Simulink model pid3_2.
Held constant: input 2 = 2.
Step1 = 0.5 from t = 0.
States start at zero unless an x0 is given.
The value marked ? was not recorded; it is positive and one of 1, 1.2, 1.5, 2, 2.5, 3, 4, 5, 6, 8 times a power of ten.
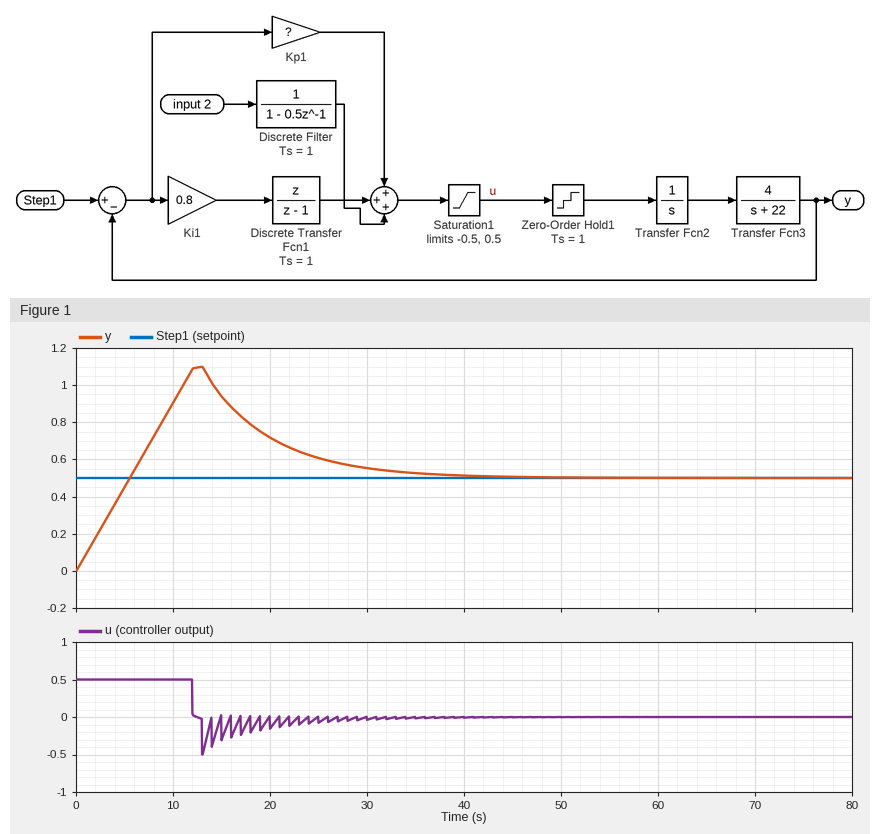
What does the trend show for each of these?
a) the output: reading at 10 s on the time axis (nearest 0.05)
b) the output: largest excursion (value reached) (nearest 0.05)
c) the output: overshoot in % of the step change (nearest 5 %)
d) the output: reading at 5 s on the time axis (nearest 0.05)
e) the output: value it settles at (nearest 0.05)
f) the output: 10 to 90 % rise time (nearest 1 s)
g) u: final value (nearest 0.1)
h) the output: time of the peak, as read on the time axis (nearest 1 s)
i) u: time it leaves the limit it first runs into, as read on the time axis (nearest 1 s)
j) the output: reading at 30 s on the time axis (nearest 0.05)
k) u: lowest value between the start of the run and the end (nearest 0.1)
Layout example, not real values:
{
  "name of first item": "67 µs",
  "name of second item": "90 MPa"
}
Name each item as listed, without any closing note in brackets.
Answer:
{
  "the output: reading at 10 s on the time axis": "0.90",
  "the output: largest excursion (value reached)": "1.10",
  "the output: overshoot in % of the step change": "120 %",
  "the output: reading at 5 s on the time axis": "0.45",
  "the output: value it settles at": "0.50",
  "the output: 10 to 90 % rise time": "4 s",
  "u: final value": "0.0",
  "the output: time of the peak, as read on the time axis": "13 s",
  "u: time it leaves the limit it first runs into, as read on the time axis": "12 s",
  "the output: reading at 30 s on the time axis": "0.55",
  "u: lowest value between the start of the run and the end": "-0.5"
}
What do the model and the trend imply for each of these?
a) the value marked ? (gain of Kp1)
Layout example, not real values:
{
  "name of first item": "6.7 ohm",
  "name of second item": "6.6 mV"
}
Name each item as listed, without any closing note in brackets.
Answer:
{
  "the value marked ?": "6"
}
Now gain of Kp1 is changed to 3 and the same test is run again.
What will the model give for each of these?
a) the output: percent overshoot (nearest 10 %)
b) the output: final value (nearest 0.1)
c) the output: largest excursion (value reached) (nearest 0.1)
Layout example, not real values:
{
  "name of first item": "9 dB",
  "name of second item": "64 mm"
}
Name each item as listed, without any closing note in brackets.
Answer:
{
  "the output: percent overshoot": "160 %",
  "the output: final value": "0.5",
  "the output: largest excursion (value reached)": "1.3"
}
